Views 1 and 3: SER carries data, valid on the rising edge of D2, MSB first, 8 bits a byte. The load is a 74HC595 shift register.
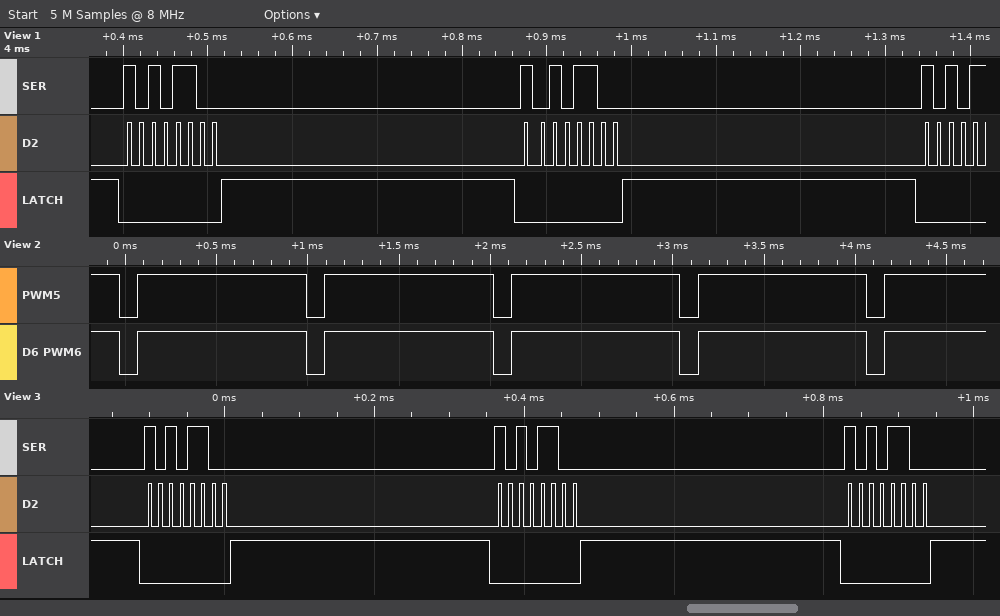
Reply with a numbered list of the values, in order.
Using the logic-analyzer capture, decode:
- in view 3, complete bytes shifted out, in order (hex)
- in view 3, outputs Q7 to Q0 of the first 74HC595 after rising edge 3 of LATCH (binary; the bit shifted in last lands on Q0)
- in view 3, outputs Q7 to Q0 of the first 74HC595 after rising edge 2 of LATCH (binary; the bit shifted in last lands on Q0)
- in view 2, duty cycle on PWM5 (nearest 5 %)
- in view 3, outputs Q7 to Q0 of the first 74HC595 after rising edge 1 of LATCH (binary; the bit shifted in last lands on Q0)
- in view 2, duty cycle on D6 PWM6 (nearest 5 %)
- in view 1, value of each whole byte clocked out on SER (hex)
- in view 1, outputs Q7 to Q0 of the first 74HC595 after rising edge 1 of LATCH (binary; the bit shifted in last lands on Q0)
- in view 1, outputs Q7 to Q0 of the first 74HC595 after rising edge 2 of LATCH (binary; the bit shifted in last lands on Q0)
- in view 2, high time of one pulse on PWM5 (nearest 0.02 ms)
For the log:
1. 0xAC 0xAC 0xAC
2. 10101100
3. 10101100
4. 90 %
5. 10101100
6. 90 %
7. AC AC
8. 10101100
9. 10101100
10. 0.92 ms
